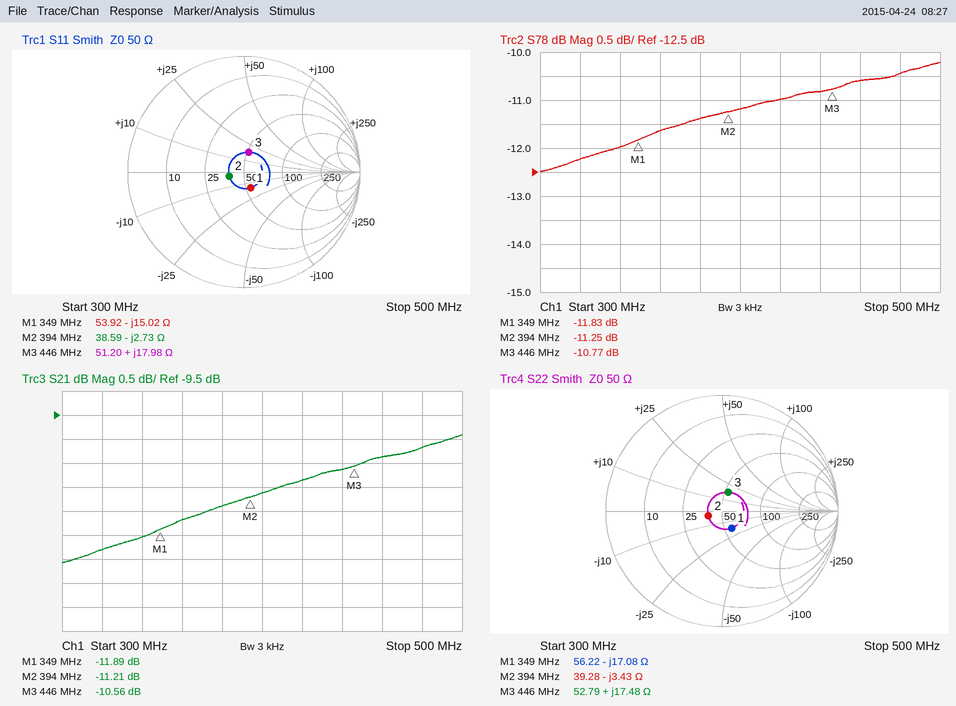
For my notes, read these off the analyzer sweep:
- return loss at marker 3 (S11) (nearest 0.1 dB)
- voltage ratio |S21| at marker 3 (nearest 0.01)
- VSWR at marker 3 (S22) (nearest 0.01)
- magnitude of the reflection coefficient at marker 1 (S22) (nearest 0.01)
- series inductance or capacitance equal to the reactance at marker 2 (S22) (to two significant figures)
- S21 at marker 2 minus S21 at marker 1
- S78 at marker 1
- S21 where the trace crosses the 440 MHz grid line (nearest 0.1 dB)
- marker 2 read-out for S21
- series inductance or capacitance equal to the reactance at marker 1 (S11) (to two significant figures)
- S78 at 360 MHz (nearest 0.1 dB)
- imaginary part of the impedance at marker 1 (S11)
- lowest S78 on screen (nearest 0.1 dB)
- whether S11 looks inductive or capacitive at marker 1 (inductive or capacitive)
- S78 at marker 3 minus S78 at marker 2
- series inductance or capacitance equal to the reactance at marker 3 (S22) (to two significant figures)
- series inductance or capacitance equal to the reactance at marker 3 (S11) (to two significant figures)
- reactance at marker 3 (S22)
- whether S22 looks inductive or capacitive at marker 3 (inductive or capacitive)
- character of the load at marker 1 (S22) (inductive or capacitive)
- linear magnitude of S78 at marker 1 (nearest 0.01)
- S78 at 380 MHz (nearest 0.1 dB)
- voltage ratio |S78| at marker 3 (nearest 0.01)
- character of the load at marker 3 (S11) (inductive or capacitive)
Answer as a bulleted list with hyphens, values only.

- 15.1 dB
- 0.30
- 1.41
- 0.17
- 120 pF
- 0.68 dB
- -11.83 dB
- -10.6 dB
- -11.21 dB
- 30 pF
- -11.6 dB
- -15.02 Ω
- -12.5 dB
- capacitive
- 0.48 dB
- 6.2 nH
- 6.4 nH
- +17.48 Ω
- inductive
- capacitive
- 0.26
- -11.4 dB
- 0.29
- inductive
